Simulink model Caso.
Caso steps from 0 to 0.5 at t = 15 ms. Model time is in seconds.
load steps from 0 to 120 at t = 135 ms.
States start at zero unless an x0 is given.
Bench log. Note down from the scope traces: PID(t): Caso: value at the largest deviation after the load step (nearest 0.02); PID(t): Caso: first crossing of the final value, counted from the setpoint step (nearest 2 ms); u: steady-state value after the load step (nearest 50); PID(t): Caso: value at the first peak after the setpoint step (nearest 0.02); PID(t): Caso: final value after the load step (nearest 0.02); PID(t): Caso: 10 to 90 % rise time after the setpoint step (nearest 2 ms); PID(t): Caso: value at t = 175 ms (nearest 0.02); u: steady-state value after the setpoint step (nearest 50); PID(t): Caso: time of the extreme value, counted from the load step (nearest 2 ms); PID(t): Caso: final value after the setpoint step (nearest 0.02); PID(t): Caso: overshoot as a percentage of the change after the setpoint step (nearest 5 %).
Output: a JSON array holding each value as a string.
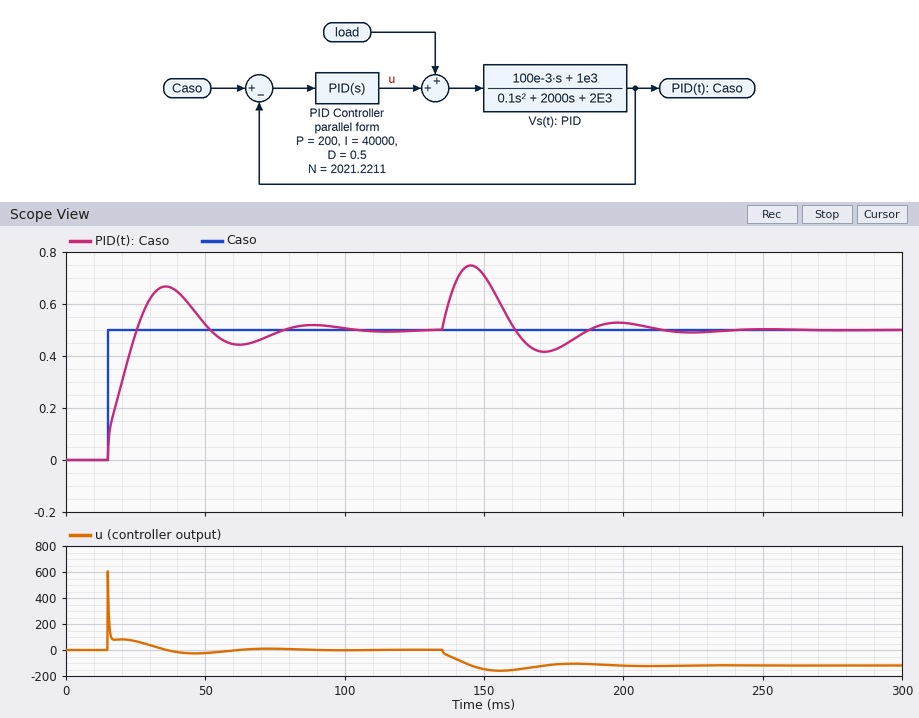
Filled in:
["0.74", "10 ms", "-100", "0.66", "0.50", "8 ms", "0.42", "0", "10 ms", "0.50", "35 %"]
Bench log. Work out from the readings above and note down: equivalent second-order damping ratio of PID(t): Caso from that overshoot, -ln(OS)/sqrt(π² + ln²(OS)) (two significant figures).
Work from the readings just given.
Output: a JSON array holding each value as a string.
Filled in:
["0.32"]
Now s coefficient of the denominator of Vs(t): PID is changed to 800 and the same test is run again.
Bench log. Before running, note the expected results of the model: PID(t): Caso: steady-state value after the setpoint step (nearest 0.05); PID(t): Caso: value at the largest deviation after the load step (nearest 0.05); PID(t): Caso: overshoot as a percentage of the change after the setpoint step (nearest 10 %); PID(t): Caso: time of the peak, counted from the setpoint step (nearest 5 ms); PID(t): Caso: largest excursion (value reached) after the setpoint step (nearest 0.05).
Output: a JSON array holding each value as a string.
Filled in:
["0.50", "0.80", "20 %", "15 ms", "0.60"]
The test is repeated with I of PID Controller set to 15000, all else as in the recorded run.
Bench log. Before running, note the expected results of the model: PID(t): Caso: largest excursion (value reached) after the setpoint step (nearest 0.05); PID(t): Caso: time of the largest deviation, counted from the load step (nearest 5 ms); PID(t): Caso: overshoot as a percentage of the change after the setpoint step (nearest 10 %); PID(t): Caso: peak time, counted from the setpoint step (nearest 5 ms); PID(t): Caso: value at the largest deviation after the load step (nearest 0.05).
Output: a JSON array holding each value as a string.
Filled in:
["0.60", "15 ms", "20 %", "30 ms", "0.85"]
